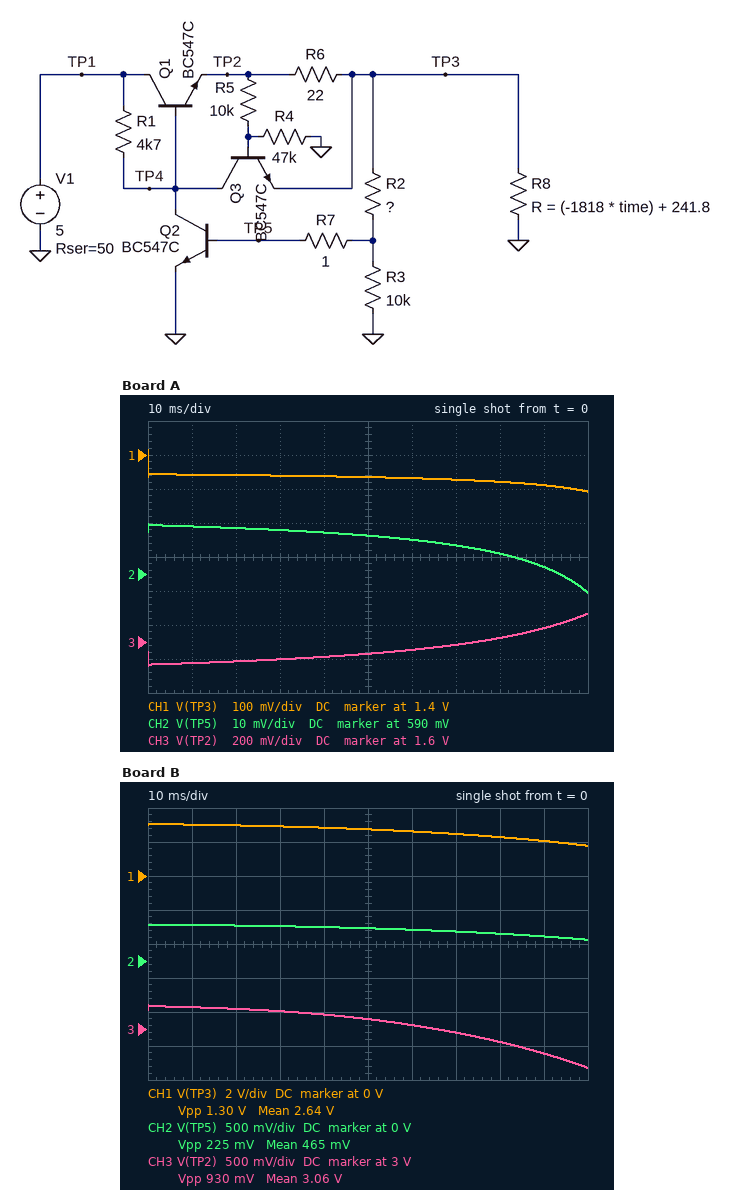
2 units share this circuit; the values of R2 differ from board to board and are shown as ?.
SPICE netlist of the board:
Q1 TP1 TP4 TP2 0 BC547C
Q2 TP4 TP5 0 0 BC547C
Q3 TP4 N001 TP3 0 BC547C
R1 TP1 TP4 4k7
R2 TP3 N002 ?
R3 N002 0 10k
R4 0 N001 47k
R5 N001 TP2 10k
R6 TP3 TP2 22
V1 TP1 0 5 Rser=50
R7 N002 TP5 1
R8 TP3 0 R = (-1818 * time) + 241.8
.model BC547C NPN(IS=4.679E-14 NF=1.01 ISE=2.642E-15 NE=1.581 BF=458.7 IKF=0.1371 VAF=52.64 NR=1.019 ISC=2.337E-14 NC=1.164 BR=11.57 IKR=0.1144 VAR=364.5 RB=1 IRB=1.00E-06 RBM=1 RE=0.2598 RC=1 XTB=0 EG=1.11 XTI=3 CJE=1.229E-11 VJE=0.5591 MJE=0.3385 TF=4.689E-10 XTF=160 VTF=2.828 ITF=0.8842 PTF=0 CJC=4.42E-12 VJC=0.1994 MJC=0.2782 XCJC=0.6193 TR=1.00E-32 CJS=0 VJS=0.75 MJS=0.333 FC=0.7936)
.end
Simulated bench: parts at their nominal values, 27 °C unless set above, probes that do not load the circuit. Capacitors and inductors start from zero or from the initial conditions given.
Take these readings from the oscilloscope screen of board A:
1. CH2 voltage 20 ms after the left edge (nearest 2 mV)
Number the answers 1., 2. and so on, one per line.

1. 604 mV
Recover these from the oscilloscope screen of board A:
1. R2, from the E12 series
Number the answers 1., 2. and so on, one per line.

1. 12 kΩ
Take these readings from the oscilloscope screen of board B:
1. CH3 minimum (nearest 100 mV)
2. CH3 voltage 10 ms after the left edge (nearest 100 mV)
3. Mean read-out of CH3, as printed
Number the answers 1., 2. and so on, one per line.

1. 2.4 V
2. 3.3 V
3. 3.06 V
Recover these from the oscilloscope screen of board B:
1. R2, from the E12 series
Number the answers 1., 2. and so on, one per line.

1. 47 kΩ
